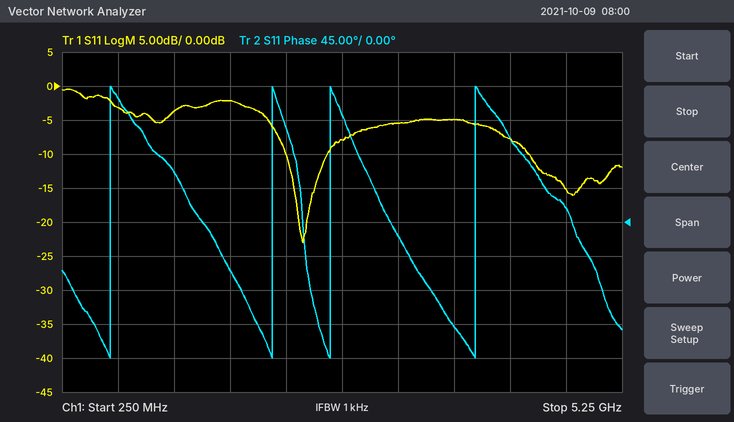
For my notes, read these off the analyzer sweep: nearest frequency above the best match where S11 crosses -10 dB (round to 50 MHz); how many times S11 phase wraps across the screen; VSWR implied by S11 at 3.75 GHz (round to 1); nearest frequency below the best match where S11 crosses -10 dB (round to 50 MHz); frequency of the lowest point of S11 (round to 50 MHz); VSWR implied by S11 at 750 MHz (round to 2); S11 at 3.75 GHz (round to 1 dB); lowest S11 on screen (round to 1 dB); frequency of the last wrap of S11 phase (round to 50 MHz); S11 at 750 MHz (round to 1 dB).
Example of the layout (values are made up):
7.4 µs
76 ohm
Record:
2.60 GHz
4
4
2.25 GHz
2.40 GHz
6
-5 dB
-23 dB
3.95 GHz
-3 dB
